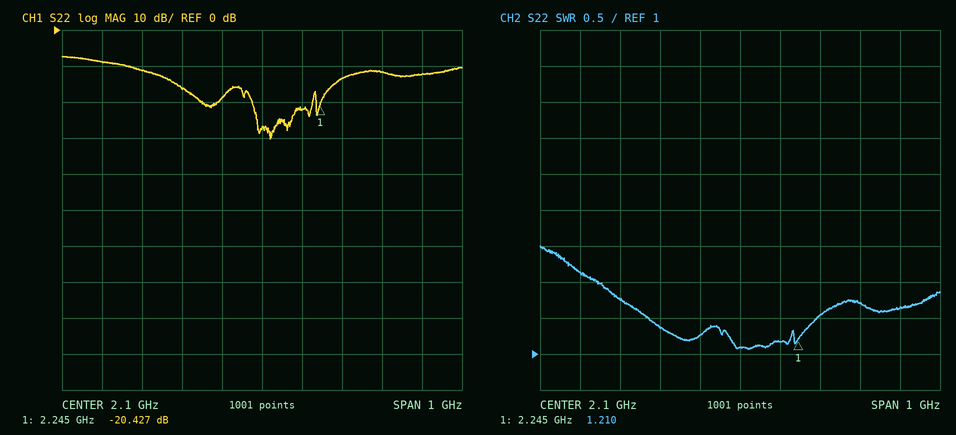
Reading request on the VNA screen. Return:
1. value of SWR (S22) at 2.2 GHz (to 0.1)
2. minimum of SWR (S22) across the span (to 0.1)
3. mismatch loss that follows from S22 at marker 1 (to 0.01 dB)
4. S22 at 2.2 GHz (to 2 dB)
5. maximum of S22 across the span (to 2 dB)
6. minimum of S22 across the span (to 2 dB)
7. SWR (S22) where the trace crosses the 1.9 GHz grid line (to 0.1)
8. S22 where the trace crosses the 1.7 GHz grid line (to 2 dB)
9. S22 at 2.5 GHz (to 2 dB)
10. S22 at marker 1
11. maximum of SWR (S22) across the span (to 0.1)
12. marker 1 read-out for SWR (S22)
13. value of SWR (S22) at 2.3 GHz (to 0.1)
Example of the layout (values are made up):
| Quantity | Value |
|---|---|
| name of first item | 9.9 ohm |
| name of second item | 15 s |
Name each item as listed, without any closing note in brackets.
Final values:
| Quantity | Value |
|---|---|
| value of SWR (S22) at 2.2 GHz | 1.2 |
| minimum of SWR (S22) across the span | 1.1 |
| mismatch loss that follows from S22 at marker 1 | 0.04 dB |
| S22 at 2.2 GHz | -22 dB |
| maximum of S22 across the span | -8 dB |
| minimum of S22 across the span | -30 dB |
| SWR (S22) where the trace crosses the 1.9 GHz grid line | 1.4 |
| S22 where the trace crosses the 1.7 GHz grid line | -8 dB |
| S22 at 2.5 GHz | -12 dB |
| S22 at marker 1 | -20.427 dB |
| maximum of SWR (S22) across the span | 2.5 |
| marker 1 read-out for SWR | 1.210 |
| value of SWR (S22) at 2.3 GHz | 1.5 |
